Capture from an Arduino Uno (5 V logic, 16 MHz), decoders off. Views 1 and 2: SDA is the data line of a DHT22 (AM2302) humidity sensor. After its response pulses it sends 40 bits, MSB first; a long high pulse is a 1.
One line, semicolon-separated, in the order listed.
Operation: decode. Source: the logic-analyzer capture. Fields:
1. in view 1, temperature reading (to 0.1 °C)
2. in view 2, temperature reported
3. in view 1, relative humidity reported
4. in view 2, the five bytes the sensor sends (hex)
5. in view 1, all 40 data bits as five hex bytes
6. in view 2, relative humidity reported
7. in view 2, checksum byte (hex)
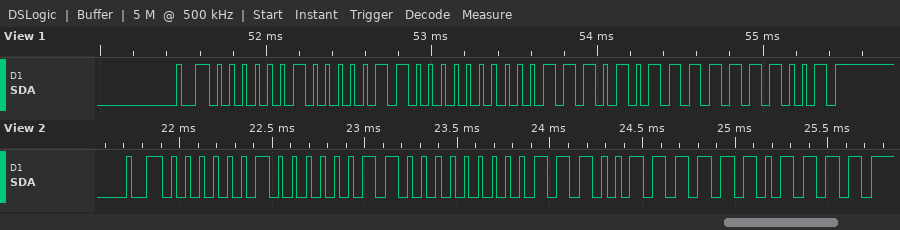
23.5 °C; 23.1 °C; 52.4 %; 02 06 00 E7 EF; 02 0C 00 EB F9; 51.8 %; 0xEF
